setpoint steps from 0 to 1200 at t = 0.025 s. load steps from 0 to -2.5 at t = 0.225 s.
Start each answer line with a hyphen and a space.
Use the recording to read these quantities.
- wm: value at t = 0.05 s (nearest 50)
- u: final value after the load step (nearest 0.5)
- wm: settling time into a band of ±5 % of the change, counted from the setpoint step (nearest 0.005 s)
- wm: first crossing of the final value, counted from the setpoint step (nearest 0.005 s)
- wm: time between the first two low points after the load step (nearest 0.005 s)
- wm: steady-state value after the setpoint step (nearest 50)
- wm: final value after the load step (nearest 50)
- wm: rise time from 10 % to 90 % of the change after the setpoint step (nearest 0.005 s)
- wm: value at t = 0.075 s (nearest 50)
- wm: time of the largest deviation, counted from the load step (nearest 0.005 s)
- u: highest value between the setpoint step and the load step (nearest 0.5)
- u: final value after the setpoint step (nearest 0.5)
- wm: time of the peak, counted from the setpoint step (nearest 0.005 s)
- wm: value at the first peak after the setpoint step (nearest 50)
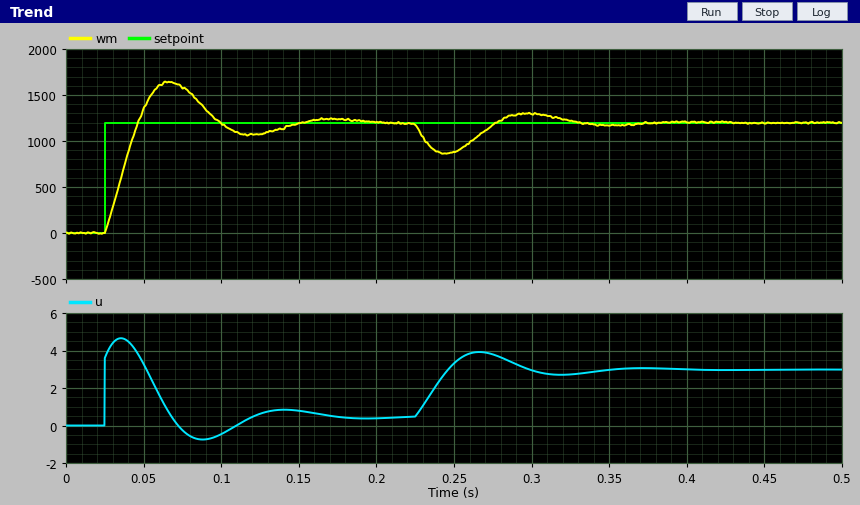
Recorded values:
- 1350
- 3.0
- 0.115 s
- 0.020 s
- 0.105 s
- 1200
- 1200
- 0.015 s
- 1600
- 0.020 s
- 4.5
- 0.5
- 0.040 s
- 1650
